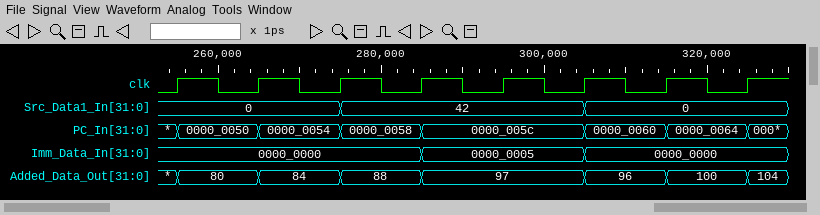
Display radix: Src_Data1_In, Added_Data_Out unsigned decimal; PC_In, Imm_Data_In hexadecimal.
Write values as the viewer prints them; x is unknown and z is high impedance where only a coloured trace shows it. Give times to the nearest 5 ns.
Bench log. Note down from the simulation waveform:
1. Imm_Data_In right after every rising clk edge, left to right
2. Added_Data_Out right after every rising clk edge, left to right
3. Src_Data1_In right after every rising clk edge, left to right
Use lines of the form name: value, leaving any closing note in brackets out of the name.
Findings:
Imm_Data_In right after every rising clk edge, left to right: 0000_0000, 0000_0000, 0000_0000, 0000_0005, 0000_0005, 0000_0000, 0000_0000, 0000_0000
Added_Data_Out right after every rising clk edge, left to right: 80, 84, 88, 97, 97, 96, 100, 104
Src_Data1_In right after every rising clk edge, left to right: 0, 0, 42, 42, 42, 0, 0, 0
